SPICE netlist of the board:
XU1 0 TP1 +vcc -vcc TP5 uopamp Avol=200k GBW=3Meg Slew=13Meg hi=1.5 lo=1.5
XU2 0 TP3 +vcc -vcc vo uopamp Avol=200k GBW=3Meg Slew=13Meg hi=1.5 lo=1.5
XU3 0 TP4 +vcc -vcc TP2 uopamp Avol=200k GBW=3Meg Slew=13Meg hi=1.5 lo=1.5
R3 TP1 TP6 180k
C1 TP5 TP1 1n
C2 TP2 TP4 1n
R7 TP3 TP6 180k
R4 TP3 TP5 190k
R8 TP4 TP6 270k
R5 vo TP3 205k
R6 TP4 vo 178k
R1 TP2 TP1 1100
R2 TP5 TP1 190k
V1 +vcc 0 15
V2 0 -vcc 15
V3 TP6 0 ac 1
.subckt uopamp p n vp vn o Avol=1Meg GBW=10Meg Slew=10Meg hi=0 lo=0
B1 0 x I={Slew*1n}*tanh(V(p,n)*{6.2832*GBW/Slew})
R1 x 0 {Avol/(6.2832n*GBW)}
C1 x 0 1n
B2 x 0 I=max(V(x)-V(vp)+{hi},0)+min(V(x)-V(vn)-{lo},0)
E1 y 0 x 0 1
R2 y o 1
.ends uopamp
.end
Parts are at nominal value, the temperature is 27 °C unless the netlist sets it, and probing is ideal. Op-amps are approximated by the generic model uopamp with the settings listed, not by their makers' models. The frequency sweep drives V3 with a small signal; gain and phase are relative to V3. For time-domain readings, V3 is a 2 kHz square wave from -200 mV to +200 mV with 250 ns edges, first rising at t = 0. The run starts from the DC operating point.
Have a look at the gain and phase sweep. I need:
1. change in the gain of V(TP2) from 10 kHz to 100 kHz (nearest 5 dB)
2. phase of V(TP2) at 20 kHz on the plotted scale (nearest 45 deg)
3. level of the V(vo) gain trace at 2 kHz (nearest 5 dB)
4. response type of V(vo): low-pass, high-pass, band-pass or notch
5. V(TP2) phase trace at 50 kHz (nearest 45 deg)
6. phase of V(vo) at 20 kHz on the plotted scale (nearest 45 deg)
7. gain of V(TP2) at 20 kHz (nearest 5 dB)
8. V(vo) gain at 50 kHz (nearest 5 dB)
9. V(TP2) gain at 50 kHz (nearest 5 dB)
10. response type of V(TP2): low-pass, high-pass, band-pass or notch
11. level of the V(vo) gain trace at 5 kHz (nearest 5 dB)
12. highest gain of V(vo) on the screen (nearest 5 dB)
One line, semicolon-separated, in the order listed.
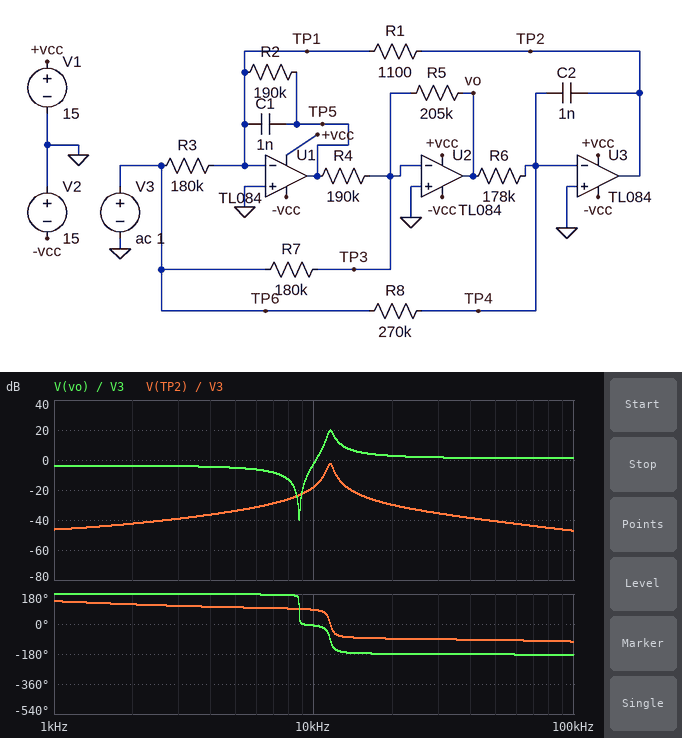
-30 dB; -90 deg; -5 dB; band-pass; -90 deg; -180 deg; -30 dB; 0 dB; -40 dB; band-pass; -5 dB; 20 dB
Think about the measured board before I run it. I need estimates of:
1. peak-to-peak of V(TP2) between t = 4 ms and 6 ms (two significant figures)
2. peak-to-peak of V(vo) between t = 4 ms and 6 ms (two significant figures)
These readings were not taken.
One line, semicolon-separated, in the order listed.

19 mV; 490 mV
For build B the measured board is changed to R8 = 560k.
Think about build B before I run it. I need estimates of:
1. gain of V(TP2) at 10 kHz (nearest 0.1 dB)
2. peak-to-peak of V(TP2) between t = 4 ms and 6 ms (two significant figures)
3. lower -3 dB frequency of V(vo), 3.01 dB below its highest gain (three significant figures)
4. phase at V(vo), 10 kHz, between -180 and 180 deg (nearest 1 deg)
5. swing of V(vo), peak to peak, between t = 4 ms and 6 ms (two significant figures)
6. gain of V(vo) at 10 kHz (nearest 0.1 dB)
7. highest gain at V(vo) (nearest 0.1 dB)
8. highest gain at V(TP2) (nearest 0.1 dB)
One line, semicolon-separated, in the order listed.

-13.2 dB; 32 mV; 11.3 kHz; -10 deg; 520 mV; 6.6 dB; 24.4 dB; 2.2 dB
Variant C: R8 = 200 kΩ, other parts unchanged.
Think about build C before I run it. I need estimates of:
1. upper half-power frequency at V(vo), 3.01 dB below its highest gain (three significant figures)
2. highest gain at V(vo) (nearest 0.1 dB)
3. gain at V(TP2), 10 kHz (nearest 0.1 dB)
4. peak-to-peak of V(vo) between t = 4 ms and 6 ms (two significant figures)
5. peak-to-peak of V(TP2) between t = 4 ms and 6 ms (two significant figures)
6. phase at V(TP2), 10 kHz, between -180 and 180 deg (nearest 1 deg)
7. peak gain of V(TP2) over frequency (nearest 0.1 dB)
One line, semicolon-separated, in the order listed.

12.0 kHz; 14.2 dB; -23.3 dB; 470 mV; 11 mV; 93 deg; -8.0 dB
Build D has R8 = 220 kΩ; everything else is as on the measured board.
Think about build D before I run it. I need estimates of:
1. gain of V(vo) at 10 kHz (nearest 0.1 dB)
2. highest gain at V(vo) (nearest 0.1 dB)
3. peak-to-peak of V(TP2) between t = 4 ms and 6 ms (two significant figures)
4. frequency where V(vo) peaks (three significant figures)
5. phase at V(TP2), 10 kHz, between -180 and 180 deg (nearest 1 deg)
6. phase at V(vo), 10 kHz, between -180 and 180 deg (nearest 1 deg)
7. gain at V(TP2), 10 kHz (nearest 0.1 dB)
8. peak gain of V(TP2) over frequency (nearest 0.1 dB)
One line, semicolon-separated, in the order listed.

-14.5 dB; 16.6 dB; 14 mV; 11.6 kHz; 89 deg; -4 deg; -21.0 dB; -5.7 dB
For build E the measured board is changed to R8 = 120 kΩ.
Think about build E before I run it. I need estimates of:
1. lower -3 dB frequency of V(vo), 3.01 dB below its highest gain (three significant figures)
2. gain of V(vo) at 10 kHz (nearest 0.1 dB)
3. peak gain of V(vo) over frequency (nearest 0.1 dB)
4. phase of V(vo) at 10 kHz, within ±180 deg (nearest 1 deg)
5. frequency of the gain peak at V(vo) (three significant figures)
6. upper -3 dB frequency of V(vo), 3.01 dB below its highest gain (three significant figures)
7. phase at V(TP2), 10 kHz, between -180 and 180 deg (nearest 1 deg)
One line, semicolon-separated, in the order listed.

11.1 kHz; 7.9 dB; 17.0 dB; 169 deg; 11.5 kHz; 11.7 kHz; -117 deg
